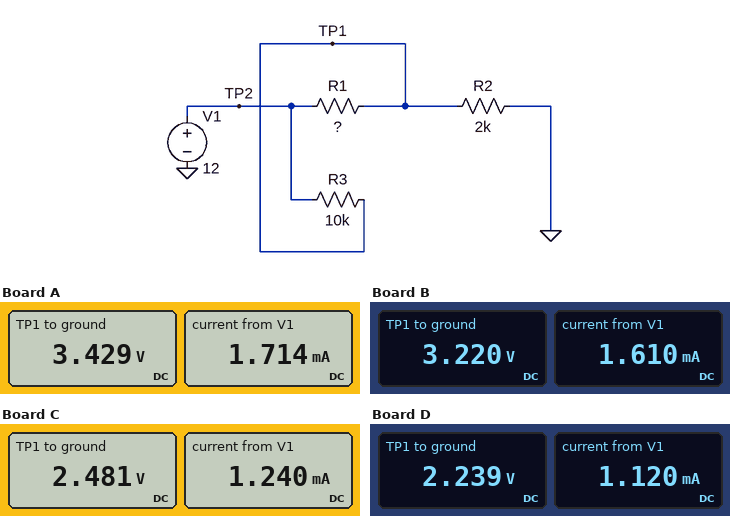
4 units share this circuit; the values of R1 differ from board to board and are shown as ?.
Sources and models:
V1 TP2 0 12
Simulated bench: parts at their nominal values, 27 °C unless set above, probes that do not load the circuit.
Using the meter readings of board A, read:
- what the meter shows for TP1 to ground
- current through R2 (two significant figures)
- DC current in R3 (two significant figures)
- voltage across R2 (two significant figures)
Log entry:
3.429 V
1.7 mA
860 µA
3.4 V
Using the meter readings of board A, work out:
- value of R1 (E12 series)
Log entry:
10 kΩ
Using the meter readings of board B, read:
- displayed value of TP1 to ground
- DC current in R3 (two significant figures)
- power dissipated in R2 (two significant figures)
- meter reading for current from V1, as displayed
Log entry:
3.220 V
880 µA
5.2 mW
1.610 mA
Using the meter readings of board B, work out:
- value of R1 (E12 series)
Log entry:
12 kΩ
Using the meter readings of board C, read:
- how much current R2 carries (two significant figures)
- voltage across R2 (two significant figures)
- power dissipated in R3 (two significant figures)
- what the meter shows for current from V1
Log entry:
1.2 mA
2.5 V
9.1 mW
1.240 mA
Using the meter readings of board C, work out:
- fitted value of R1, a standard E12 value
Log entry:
33 kΩ
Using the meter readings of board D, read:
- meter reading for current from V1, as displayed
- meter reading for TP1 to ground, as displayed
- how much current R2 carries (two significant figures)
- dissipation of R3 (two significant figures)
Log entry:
1.120 mA
2.239 V
1.1 mA
9.5 mW
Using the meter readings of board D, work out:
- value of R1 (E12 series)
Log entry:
68 kΩ
